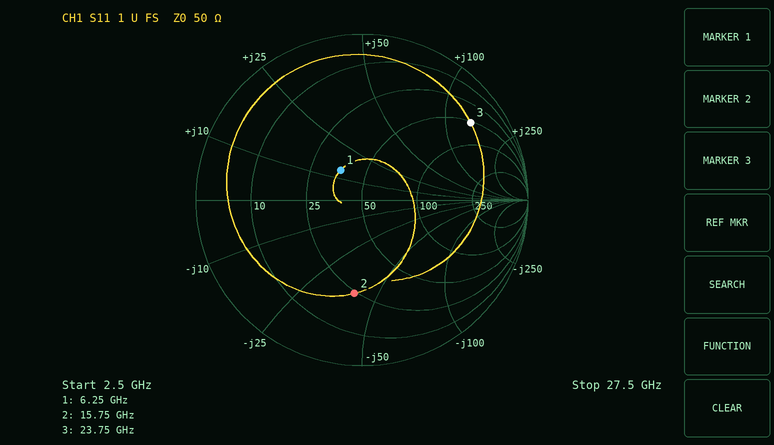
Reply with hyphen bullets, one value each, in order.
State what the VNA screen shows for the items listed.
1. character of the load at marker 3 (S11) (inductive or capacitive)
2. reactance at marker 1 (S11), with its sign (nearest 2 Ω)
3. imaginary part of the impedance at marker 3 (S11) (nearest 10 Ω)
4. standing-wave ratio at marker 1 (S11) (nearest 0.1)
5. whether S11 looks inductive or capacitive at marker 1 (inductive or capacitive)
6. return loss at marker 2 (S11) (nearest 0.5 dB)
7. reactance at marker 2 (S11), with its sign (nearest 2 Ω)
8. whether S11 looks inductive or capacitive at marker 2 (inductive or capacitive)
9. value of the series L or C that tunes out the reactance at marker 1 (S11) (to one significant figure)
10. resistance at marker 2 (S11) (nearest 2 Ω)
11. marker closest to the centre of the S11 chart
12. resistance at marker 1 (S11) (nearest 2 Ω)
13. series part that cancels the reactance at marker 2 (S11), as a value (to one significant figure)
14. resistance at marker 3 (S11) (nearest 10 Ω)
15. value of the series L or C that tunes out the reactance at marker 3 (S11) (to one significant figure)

- inductive
- +14 Ω
- +140 Ω
- 1.6
- inductive
- 5.0 dB
- -40 Ω
- capacitive
- 2 pF
- 24 Ω
- marker 1
- 36 Ω
- 400 pH
- 50 Ω
- 50 fF
